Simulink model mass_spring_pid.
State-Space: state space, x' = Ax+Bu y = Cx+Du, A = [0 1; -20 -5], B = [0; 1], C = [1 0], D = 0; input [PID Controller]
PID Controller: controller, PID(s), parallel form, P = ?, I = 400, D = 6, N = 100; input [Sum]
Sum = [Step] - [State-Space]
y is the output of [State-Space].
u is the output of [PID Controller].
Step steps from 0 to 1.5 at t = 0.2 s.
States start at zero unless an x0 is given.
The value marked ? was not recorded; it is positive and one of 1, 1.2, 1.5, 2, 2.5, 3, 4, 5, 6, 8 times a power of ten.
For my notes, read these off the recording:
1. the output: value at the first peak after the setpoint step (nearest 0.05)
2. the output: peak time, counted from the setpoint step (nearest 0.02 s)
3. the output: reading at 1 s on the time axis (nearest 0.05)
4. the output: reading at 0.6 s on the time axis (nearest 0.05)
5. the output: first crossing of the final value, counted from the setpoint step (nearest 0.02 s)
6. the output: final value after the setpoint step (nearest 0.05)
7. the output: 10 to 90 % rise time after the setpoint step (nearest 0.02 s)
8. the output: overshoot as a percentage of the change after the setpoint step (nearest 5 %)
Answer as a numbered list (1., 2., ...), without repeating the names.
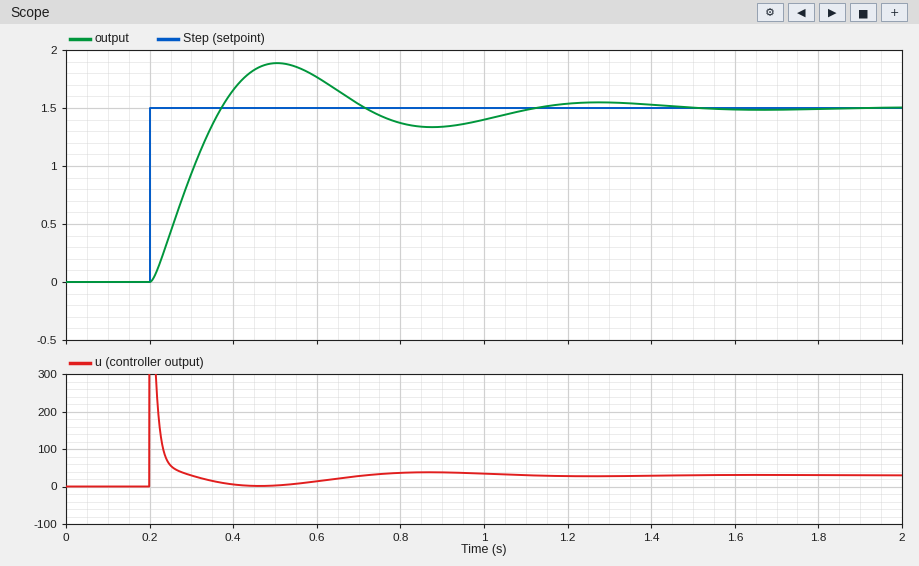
1. 1.90
2. 0.30 s
3. 1.40
4. 1.75
5. 0.18 s
6. 1.50
7. 0.12 s
8. 25 %
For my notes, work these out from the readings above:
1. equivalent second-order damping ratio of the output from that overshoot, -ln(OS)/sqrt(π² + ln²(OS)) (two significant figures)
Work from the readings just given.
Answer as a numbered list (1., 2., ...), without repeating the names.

1. 0.40
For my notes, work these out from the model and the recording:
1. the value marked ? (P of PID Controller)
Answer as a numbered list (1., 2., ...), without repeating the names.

1. 80
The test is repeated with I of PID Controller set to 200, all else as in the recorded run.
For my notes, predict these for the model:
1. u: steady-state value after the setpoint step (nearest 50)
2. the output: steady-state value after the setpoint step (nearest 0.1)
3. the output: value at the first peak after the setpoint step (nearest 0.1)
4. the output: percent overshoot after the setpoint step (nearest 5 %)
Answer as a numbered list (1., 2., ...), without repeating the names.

1. 50
2. 1.5
3. 1.7
4. 10 %
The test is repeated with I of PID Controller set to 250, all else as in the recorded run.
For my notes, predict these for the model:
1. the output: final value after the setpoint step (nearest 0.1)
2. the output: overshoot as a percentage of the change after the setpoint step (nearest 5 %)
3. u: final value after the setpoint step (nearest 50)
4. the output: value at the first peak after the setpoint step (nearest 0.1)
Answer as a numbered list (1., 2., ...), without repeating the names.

1. 1.5
2. 15 %
3. 50
4. 1.7
